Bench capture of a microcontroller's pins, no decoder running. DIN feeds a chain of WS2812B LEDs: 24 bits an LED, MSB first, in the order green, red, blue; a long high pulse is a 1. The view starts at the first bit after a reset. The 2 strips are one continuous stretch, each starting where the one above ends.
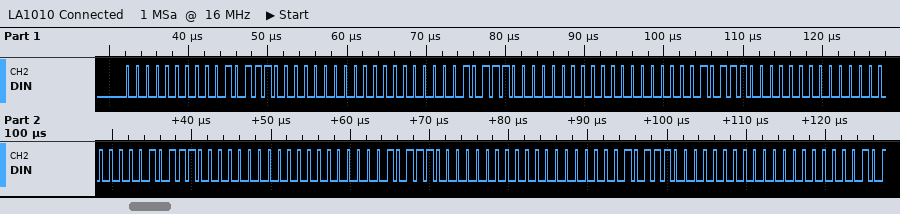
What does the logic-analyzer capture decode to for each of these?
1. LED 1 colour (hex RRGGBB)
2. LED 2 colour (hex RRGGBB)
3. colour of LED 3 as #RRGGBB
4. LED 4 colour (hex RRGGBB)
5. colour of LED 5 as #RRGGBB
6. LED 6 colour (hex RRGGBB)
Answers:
#2E0000
#2E0000
#2E0000
#2E0000
#2E0000
#2E0000
